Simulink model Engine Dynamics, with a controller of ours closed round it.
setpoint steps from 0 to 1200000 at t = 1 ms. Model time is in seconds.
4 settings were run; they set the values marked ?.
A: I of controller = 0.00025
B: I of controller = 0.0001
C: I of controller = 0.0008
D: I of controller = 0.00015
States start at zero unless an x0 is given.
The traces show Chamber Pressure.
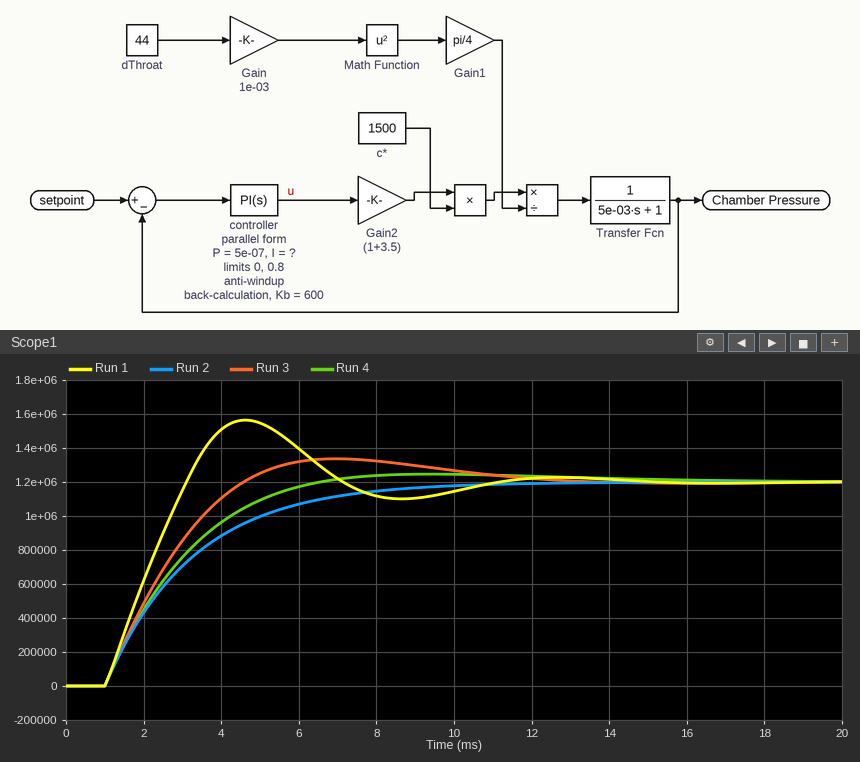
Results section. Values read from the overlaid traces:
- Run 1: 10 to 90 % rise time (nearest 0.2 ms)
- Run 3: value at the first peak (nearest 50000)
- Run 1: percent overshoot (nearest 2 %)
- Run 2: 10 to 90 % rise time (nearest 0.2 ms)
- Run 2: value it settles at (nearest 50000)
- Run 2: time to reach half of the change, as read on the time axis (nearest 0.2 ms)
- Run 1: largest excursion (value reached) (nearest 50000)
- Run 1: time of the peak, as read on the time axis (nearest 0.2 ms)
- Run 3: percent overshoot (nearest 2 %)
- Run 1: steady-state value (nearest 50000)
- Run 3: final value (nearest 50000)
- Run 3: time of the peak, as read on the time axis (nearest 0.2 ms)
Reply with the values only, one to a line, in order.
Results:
1.6 ms
1350000
30 %
5.0 ms
1200000
2.6 ms
1550000
4.6 ms
12 %
1200000
1200000
7.0 ms
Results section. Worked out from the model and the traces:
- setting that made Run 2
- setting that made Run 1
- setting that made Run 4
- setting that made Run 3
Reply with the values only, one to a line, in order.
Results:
B
C
D
A
